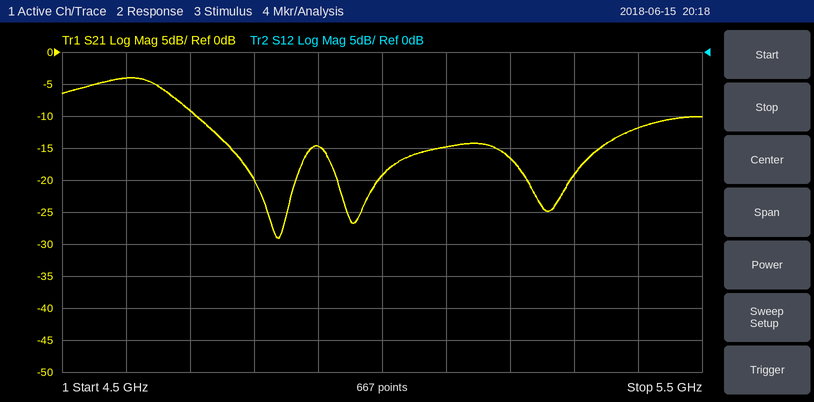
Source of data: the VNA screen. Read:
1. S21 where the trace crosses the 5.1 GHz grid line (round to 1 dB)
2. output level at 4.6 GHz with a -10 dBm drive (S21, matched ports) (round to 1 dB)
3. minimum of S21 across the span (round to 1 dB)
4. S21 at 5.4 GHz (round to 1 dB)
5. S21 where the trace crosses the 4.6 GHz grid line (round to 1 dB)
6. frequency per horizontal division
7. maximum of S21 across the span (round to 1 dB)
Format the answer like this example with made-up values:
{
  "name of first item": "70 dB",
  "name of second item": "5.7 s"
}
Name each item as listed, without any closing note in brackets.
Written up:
{
  "S21 where the trace crosses the 5.1 GHz grid line": "-15 dB",
  "output level at 4.6 GHz with a -10 dBm drive (S21, matched ports)": "-14 dBm",
  "minimum of S21 across the span": "-29 dB",
  "S21 at 5.4 GHz": "-12 dB",
  "S21 where the trace crosses the 4.6 GHz grid line": "-4 dB",
  "frequency per horizontal division": "100 MHz",
  "maximum of S21 across the span": "-4 dB"
}
